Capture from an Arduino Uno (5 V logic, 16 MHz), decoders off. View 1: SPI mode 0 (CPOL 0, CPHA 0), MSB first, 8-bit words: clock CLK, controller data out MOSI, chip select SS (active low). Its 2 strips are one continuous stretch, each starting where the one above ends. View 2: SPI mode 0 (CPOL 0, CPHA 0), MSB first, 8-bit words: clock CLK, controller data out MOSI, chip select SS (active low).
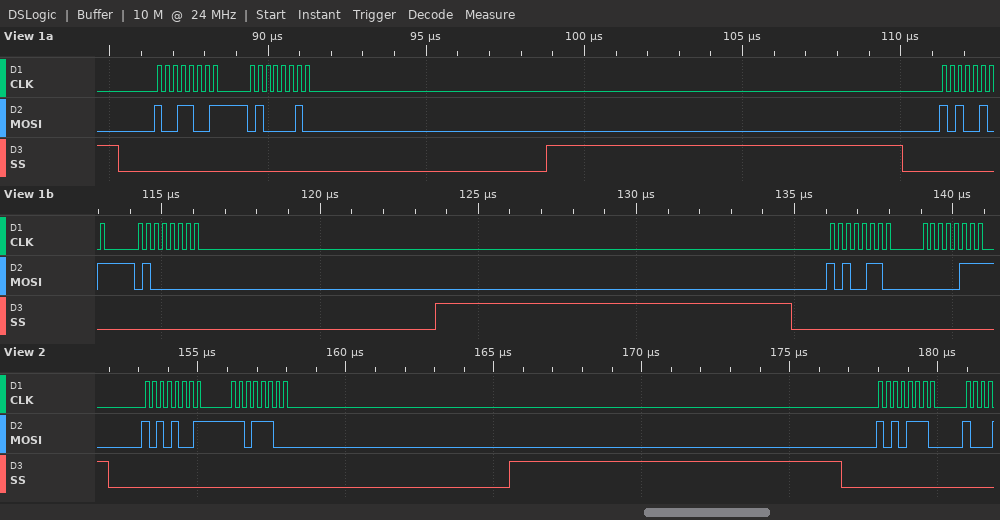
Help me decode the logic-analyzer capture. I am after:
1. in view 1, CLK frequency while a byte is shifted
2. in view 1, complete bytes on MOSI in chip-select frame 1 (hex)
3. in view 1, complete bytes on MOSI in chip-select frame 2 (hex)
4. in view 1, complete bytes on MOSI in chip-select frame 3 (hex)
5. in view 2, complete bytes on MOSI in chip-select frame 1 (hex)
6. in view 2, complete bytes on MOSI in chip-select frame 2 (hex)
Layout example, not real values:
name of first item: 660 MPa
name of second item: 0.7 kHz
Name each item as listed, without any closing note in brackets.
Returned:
in view 1, CLK frequency while a byte is shifted: 4 MHz
in view 1, complete bytes on MOSI in chip-select frame 1: 0x99 0x42
in view 1, complete bytes on MOSI in chip-select frame 2: 0xA5 0x40
in view 1, complete bytes on MOSI in chip-select frame 3: 0xA6 0x07
in view 2, complete bytes on MOSI in chip-select frame 1: A9 DC
in view 2, complete bytes on MOSI in chip-select frame 2: AE
